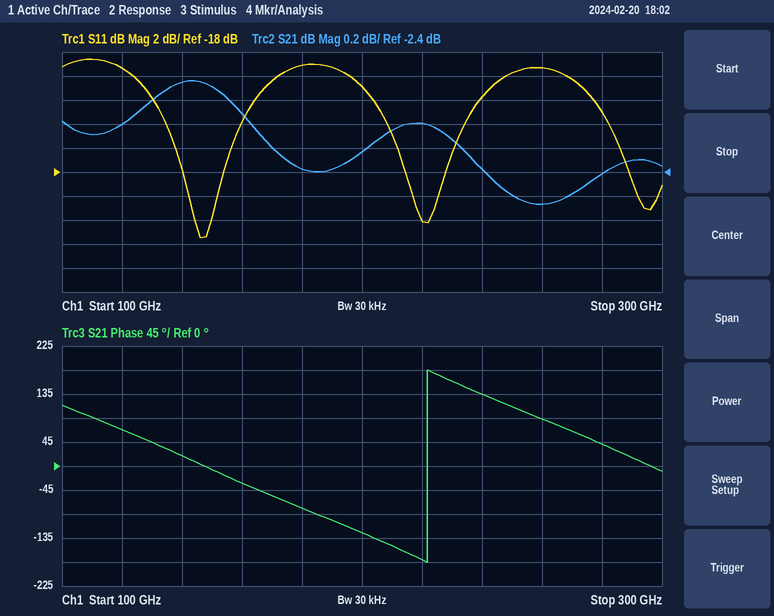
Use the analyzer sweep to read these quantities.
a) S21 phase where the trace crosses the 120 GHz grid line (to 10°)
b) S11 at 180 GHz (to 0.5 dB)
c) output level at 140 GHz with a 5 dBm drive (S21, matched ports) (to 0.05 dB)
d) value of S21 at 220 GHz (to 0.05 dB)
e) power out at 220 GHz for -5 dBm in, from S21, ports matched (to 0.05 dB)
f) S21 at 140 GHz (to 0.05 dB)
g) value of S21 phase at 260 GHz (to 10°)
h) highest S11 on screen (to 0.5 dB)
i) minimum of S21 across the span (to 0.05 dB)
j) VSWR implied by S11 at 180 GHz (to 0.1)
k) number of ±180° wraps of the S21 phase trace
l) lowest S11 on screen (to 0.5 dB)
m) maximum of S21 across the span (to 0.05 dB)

70°
-9.0 dB
3.35 dBm
-2.00 dB
-7.00 dBm
-1.65 dB
90°
-8.5 dB
-2.65 dB
2.1
1
-23.5 dB
-1.65 dB
